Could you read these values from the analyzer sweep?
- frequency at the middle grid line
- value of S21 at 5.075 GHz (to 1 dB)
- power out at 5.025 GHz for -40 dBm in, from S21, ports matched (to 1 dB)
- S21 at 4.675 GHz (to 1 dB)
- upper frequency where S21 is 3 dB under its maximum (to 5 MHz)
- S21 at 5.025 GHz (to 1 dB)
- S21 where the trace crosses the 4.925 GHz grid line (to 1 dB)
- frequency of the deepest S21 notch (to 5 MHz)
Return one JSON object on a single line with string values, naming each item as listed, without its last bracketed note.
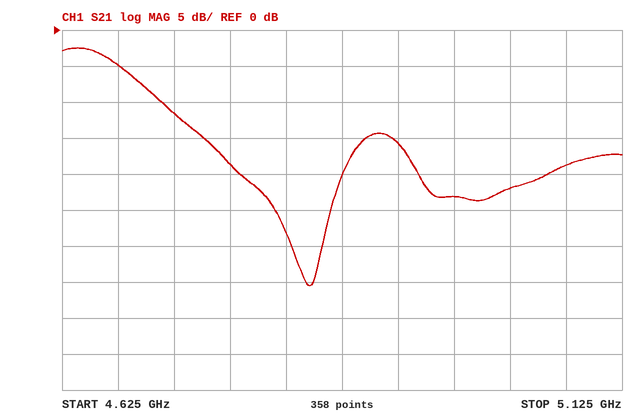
{"frequency at the middle grid line": "4.875 GHz", "value of S21 at 5.075 GHz": "-19 dB", "power out at 5.025 GHz for -40 dBm in, from S21, ports matched": "-62 dBm", "S21 at 4.675 GHz": "-5 dB", "upper frequency where S21 is 3 dB under its maximum": "4.680 GHz", "S21 at 5.025 GHz": "-22 dB", "S21 where the trace crosses the 4.925 GHz grid line": "-16 dB", "frequency of the deepest S21 notch": "4.845 GHz"}
